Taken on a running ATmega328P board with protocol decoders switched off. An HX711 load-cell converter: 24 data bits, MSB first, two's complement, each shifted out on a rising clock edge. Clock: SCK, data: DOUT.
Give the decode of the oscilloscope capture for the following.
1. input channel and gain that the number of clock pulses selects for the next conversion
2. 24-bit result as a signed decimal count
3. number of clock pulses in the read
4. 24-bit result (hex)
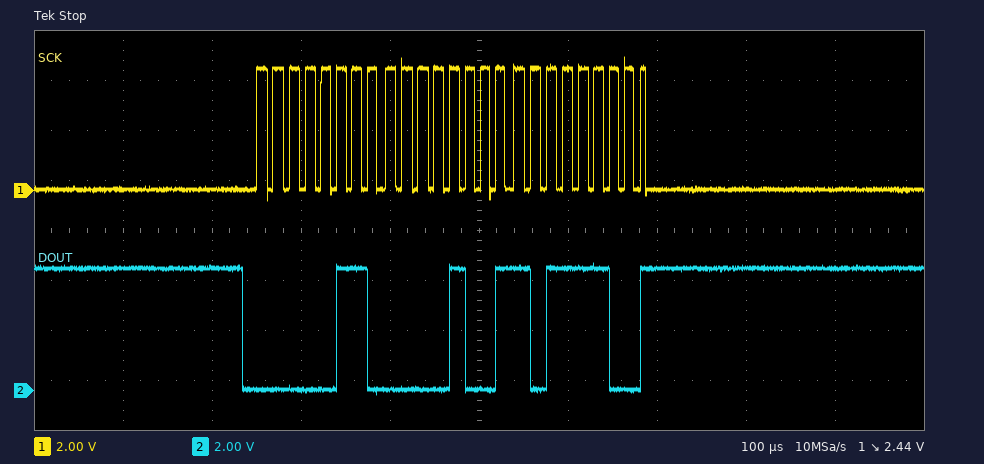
channel A, gain 128
395708
25
0x0609BC
